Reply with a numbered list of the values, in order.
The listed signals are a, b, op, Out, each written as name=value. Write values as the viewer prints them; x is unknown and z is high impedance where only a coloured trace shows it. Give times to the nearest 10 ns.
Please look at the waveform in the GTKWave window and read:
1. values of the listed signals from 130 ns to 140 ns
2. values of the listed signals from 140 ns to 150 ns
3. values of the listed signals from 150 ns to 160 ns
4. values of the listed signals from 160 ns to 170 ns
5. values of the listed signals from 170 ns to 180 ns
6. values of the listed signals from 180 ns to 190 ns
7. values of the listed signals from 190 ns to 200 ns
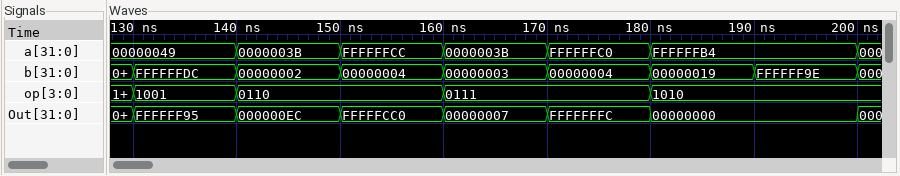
1. a=00000049, b=FFFFFFDC, op=1001, Out=FFFFFF95
2. a=0000003B, b=00000002, op=0110, Out=000000EC
3. a=FFFFFFCC, b=00000004, op=0110, Out=FFFFFCC0
4. a=0000003B, b=00000003, op=0111, Out=00000007
5. a=FFFFFFC0, b=00000004, op=0111, Out=FFFFFFFC
6. a=FFFFFFB4, b=00000019, op=1010, Out=00000000
7. a=FFFFFFB4, b=FFFFFF9E, op=1010, Out=00000000
